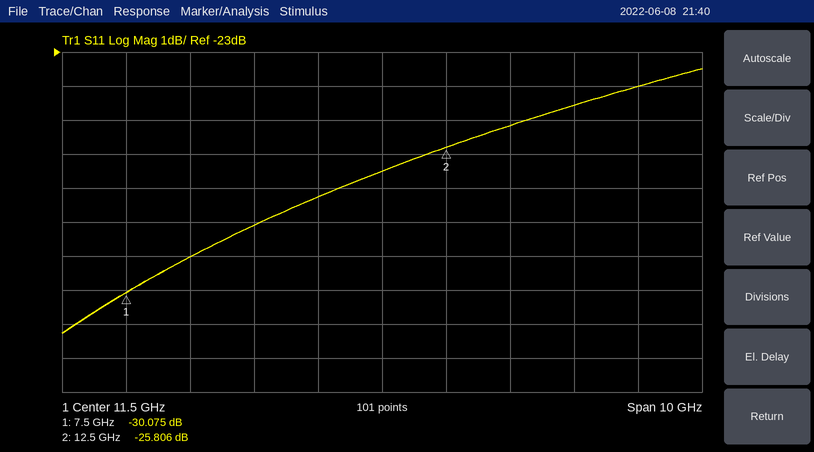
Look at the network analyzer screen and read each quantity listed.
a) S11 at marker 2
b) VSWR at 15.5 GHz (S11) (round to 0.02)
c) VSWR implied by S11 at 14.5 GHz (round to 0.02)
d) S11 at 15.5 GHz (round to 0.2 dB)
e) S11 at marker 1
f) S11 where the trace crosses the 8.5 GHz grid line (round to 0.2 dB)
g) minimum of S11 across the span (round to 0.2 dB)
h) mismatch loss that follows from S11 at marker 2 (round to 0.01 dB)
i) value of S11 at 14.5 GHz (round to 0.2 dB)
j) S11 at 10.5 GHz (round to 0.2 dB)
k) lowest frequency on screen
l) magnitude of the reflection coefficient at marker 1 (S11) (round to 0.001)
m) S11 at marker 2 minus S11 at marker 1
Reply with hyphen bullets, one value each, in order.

- -25.806 dB
- 1.14
- 1.12
- -24.0 dB
- -30.075 dB
- -29.0 dB
- -31.2 dB
- 0.01 dB
- -24.6 dB
- -27.2 dB
- 6.5 GHz
- 0.031
- 4.269 dB
